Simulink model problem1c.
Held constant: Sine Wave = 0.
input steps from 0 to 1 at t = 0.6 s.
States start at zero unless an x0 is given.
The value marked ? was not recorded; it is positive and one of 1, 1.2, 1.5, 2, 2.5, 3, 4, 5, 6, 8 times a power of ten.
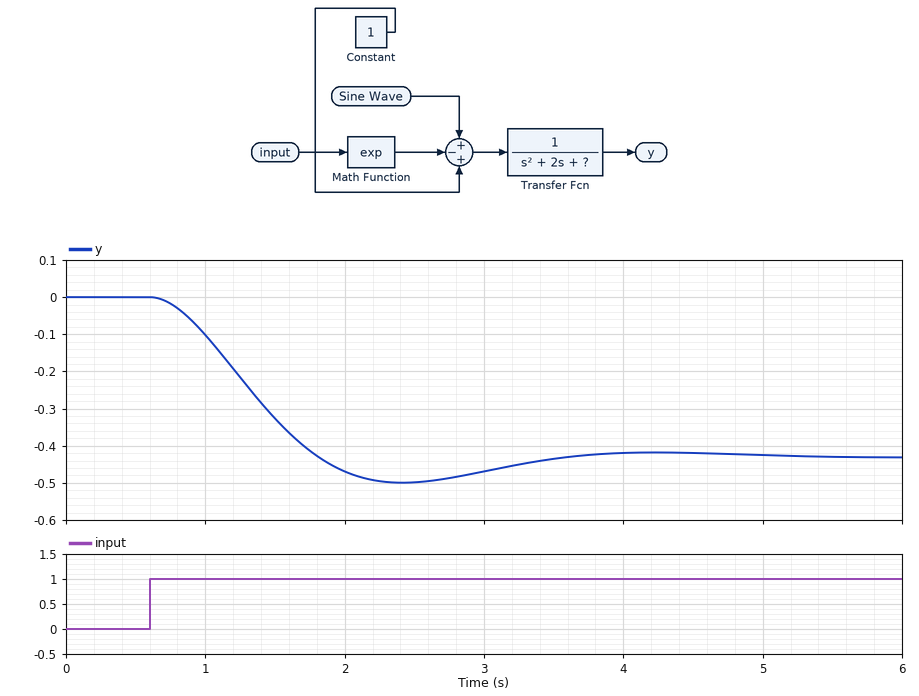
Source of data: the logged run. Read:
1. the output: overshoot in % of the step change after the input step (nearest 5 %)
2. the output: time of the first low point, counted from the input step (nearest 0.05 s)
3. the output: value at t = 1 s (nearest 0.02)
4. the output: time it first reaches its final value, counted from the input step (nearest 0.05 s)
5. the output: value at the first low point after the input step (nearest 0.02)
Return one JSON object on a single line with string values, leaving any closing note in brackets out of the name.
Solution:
{"the output: overshoot in % of the step change after the input step": "15 %", "the output: time of the first low point, counted from the input step": "1.80 s", "the output: value at t = 1 s": "-0.10", "the output: time it first reaches its final value, counted from the input step": "1.20 s", "the output: value at the first low point after the input step": "-0.50"}
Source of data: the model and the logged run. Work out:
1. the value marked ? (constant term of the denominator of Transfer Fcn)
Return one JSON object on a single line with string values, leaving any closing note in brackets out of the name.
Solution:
{"the value marked ?": "4"}
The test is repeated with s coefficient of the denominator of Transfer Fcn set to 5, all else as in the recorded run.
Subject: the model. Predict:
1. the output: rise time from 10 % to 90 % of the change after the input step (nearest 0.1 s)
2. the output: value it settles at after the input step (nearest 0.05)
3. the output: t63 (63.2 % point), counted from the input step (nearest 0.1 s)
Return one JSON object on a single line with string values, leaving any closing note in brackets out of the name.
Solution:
{"the output: rise time from 10 % to 90 % of the change after the input step": "2.3 s", "the output: value it settles at after the input step": "-0.45", "the output: t63 (63.2 % point), counted from the input step": "1.3 s"}
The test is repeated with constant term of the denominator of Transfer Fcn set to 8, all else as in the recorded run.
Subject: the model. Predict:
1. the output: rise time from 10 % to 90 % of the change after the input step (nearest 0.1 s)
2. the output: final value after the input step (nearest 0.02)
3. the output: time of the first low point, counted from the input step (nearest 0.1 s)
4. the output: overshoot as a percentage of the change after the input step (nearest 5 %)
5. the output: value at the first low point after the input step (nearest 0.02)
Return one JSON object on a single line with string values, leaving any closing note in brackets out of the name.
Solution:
{"the output: rise time from 10 % to 90 % of the change after the input step": "0.5 s", "the output: final value after the input step": "-0.22", "the output: time of the first low point, counted from the input step": "1.2 s", "the output: overshoot as a percentage of the change after the input step": "30 %", "the output: value at the first low point after the input step": "-0.28"}
